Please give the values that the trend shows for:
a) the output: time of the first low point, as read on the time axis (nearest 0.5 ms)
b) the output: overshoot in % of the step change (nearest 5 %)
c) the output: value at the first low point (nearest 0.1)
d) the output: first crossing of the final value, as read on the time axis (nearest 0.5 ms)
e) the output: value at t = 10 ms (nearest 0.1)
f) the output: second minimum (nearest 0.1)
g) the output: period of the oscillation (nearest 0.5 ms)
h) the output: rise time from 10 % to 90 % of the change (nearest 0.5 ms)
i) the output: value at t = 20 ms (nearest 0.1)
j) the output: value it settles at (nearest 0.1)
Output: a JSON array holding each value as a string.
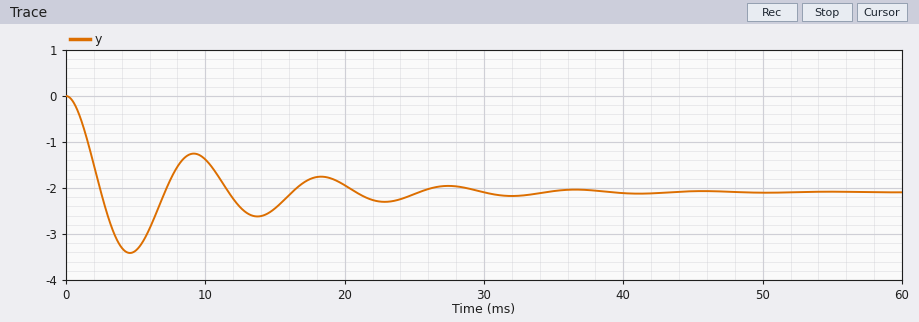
["4.5 ms", "65 %", "-3.4", "2.5 ms", "-1.4", "-2.6", "9.0 ms", "1.5 ms", "-1.9", "-2.1"]
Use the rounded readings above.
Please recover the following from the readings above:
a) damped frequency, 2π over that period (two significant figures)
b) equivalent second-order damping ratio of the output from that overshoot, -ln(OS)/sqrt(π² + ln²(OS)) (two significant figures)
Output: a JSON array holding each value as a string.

["0.70 rad/ms", "0.14"]
